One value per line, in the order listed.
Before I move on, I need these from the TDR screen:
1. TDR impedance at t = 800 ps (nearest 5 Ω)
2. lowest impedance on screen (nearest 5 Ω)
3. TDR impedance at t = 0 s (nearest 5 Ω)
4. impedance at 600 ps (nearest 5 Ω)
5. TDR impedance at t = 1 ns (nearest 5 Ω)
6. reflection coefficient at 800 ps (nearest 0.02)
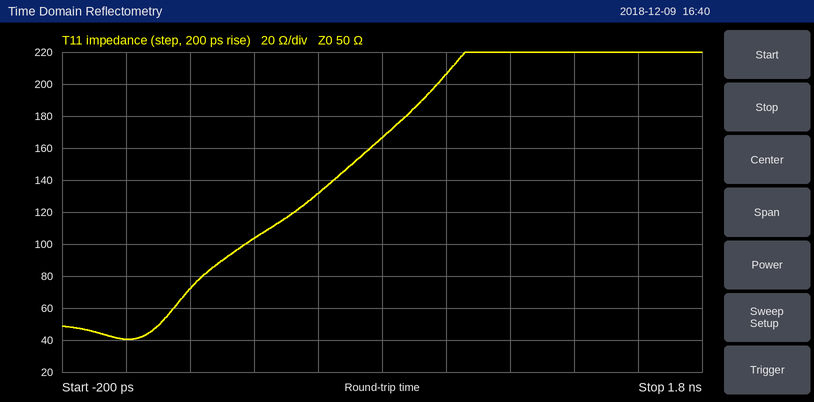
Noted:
165 Ω
40 Ω
40 Ω
130 Ω
205 Ω
+0.54
